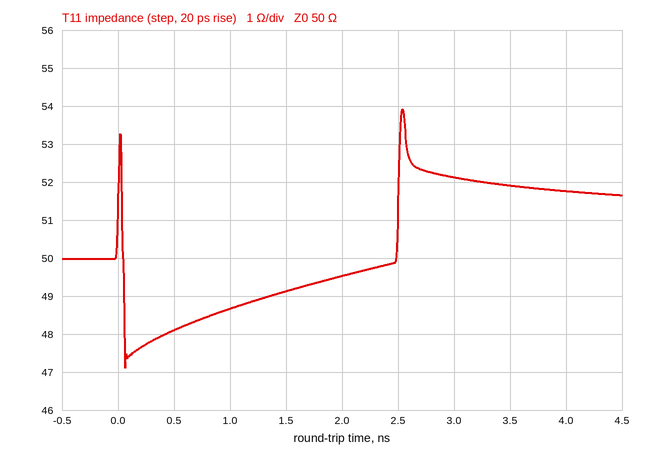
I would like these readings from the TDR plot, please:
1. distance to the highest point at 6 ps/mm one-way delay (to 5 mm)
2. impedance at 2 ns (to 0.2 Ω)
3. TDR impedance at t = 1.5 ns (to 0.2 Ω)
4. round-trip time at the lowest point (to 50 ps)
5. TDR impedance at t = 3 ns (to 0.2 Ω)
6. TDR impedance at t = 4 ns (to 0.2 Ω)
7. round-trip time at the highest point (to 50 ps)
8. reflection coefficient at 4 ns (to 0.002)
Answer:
210 mm
49.6 Ω
49.2 Ω
50 ps
52.2 Ω
51.8 Ω
2.55 ns
+0.018
